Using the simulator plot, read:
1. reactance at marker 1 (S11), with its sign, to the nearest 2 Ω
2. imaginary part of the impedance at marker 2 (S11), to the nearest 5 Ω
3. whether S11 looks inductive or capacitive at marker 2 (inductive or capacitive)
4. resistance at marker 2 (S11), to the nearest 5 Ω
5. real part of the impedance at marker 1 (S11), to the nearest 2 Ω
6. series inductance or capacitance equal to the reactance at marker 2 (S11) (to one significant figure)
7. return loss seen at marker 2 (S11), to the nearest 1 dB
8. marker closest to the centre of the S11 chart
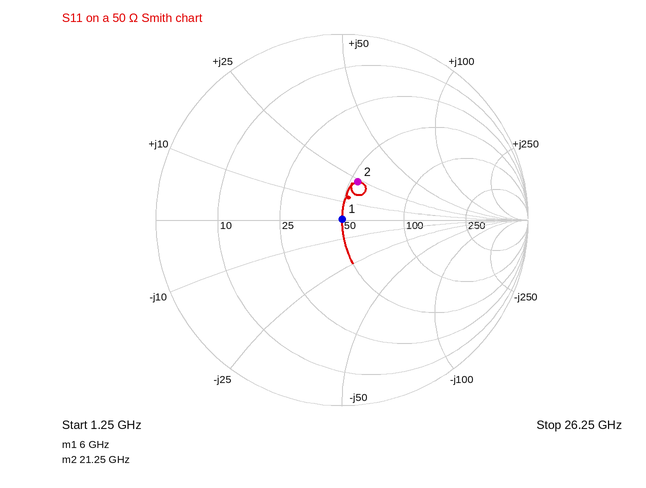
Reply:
0 Ω
+25 Ω
inductive
55 Ω
50 Ω
200 pH
13 dB
marker 1
